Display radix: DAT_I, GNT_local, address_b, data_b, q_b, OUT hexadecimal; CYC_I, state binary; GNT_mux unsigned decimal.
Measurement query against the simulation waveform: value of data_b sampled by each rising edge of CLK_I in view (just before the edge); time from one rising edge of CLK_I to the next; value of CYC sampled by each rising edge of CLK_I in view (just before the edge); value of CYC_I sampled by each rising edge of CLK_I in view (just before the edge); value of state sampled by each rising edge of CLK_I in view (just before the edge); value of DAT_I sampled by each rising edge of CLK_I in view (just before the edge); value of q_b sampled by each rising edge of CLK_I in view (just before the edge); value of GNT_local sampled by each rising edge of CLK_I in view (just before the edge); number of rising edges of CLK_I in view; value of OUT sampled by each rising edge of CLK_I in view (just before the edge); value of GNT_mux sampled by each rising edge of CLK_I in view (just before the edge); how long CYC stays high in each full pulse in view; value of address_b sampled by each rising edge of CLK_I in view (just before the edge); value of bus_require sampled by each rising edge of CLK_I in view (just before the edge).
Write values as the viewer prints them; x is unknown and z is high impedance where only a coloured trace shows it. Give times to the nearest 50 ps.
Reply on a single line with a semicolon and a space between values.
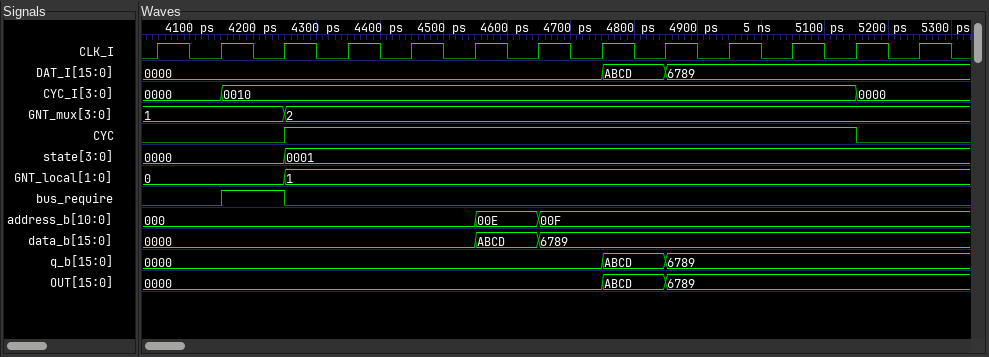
0000, 0000, 0000, 0000, 0000, 0000, ABCD, 6789, 6789, 6789, 6789, 6789, 6789; 100 ps; 0 0 0 1 1 1 1 1 1 1 1 1 0; 0000, 0000, 0010, 0010, 0010, 0010, 0010, 0010, 0010, 0010, 0010, 0010, 0000; 0000, 0000, 0000, 0001, 0001, 0001, 0001, 0001, 0001, 0001, 0001, 0001, 0001; 0000, 0000, 0000, 0000, 0000, 0000, 0000, 0000, ABCD, 6789, 6789, 6789, 6789; 0000, 0000, 0000, 0000, 0000, 0000, 0000, 0000, ABCD, 6789, 6789, 6789, 6789; 0, 0, 0, 1, 1, 1, 1, 1, 1, 1, 1, 1, 1; 13; 0000, 0000, 0000, 0000, 0000, 0000, 0000, 0000, ABCD, 6789, 6789, 6789, 6789; 1, 1, 1, 2, 2, 2, 2, 2, 2, 2, 2, 2, 2; 900 ps; 000, 000, 000, 000, 000, 000, 00E, 00F, 00F, 00F, 00F, 00F, 00F; 0 0 1 0 0 0 0 0 0 0 0 0 0
